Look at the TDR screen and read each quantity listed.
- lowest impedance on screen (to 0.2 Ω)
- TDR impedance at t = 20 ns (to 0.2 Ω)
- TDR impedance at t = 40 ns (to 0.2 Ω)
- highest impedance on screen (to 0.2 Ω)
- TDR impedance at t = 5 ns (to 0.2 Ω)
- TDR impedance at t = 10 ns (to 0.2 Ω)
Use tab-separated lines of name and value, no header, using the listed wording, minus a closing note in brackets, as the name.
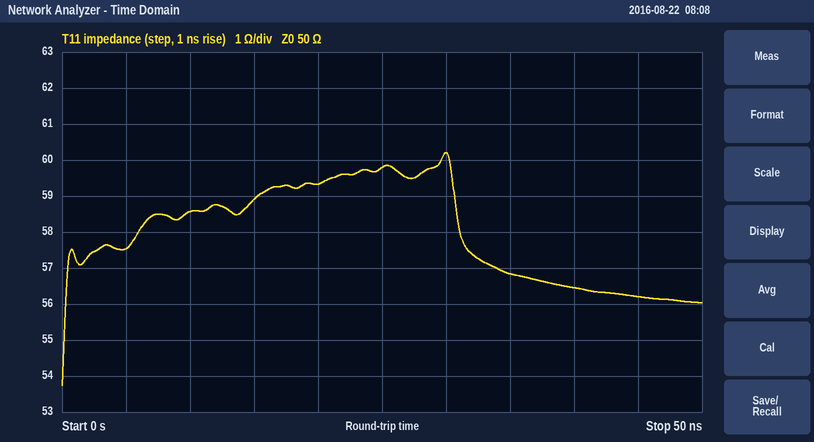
lowest impedance on screen	53.8 Ω
TDR impedance at t = 20 ns	59.4 Ω
TDR impedance at t = 40 ns	56.4 Ω
highest impedance on screen	60.2 Ω
TDR impedance at t = 5 ns	57.6 Ω
TDR impedance at t = 10 ns	58.6 Ω
